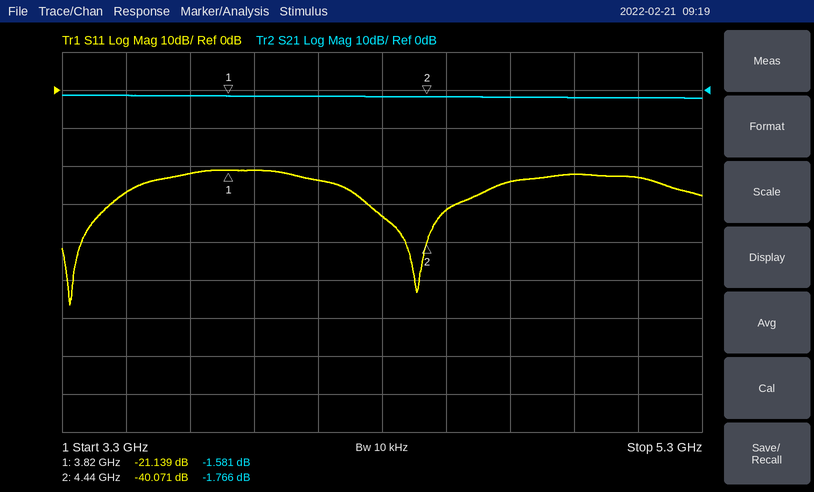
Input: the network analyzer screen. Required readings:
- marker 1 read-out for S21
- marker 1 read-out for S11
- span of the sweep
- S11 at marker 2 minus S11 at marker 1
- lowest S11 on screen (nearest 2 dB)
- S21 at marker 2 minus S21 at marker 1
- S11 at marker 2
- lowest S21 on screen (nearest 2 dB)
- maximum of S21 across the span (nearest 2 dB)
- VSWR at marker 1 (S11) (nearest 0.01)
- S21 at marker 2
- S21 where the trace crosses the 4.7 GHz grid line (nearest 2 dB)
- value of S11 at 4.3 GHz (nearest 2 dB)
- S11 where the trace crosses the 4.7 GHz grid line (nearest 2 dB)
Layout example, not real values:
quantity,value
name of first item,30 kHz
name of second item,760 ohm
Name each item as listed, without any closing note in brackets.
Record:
quantity,value
marker 1 read-out for S21,-1.581 dB
marker 1 read-out for S11,-21.139 dB
span of the sweep,2 GHz
S11 at marker 2 minus S11 at marker 1,-18.932 dB
lowest S11 on screen,-56 dB
S21 at marker 2 minus S21 at marker 1,-0.185 dB
S11 at marker 2,-40.071 dB
lowest S21 on screen,-2 dB
maximum of S21 across the span,-2 dB
VSWR at marker 1 (S11),1.19
S21 at marker 2,-1.766 dB
S21 where the trace crosses the 4.7 GHz grid line,-2 dB
value of S11 at 4.3 GHz,-34 dB
S11 where the trace crosses the 4.7 GHz grid line,-24 dB
